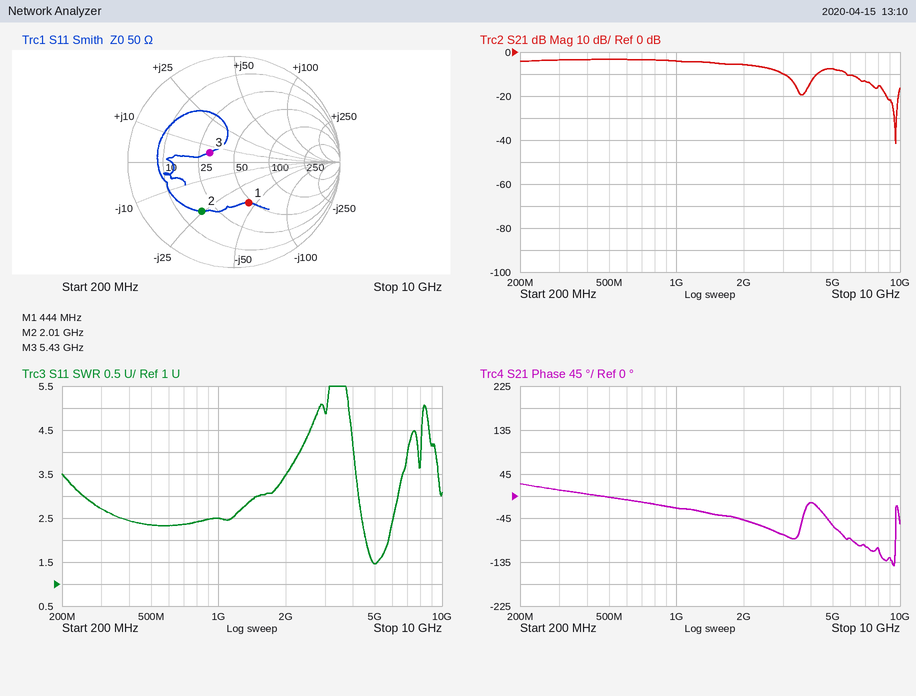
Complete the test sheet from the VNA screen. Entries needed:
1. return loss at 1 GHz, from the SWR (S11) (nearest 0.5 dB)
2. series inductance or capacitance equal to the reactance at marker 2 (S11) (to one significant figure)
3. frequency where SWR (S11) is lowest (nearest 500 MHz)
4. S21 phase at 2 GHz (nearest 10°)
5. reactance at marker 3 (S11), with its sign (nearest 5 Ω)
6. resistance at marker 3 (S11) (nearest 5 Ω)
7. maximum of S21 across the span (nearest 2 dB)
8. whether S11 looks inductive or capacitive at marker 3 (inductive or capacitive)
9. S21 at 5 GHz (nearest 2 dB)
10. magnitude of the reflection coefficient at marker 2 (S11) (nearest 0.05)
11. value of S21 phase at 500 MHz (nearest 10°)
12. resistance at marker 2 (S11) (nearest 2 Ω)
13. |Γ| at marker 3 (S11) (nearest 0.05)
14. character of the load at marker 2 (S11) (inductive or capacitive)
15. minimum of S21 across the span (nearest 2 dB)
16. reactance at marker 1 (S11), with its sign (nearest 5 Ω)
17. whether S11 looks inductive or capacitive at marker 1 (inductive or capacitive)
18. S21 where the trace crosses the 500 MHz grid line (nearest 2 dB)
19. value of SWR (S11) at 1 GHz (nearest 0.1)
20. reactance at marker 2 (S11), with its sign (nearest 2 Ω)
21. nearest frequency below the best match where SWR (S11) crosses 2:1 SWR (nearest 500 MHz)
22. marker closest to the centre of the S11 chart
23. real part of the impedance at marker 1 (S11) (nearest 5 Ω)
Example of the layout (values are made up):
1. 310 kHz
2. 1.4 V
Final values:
1. 7.5 dB
2. 3 pF
3. 5.0 GHz
4. -50°
5. +5 Ω
6. 30 Ω
7. -4 dB
8. inductive
9. -8 dB
10. 0.55
11. 0°
12. 18 Ω
13. 0.25
14. capacitive
15. -42 dB
16. -45 Ω
17. capacitive
18. -4 dB
19. 2.5
20. -24 Ω
21. 4.5 GHz
22. marker 3
23. 45 Ω
